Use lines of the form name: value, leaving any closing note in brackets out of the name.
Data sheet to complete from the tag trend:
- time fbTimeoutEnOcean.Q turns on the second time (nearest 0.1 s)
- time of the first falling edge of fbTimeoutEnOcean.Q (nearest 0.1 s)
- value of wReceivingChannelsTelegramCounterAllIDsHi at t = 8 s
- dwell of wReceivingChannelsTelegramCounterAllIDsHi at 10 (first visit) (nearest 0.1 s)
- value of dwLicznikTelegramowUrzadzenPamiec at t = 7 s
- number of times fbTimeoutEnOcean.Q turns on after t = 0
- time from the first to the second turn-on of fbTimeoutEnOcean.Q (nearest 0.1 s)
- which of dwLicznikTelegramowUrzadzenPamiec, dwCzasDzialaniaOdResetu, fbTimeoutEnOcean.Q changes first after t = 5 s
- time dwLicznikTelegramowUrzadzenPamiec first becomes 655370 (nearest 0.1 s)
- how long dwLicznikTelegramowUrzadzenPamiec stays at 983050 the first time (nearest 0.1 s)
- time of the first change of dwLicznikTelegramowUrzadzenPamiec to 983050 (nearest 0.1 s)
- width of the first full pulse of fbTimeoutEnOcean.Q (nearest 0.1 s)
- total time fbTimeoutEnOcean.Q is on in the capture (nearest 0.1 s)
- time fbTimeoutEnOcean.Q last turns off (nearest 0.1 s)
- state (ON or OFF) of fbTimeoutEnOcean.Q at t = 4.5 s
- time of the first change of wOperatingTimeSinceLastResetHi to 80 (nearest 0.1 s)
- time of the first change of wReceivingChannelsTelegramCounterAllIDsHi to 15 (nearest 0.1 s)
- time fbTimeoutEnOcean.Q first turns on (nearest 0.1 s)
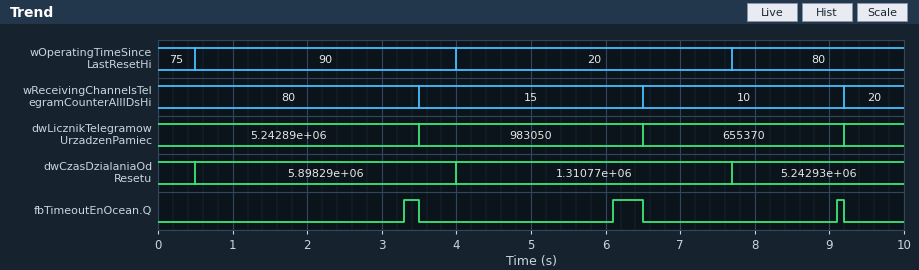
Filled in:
time fbTimeoutEnOcean.Q turns on the second time: 6.1 s
time of the first falling edge of fbTimeoutEnOcean.Q: 3.5 s
value of wReceivingChannelsTelegramCounterAllIDsHi at t = 8 s: 10
dwell of wReceivingChannelsTelegramCounterAllIDsHi at 10 (first visit): 2.7 s
value of dwLicznikTelegramowUrzadzenPamiec at t = 7 s: 655370
number of times fbTimeoutEnOcean.Q turns on after t = 0: 3
time from the first to the second turn-on of fbTimeoutEnOcean.Q: 2.8 s
which of dwLicznikTelegramowUrzadzenPamiec, dwCzasDzialaniaOdResetu, fbTimeoutEnOcean.Q changes first after t = 5 s: fbTimeoutEnOcean.Q
time dwLicznikTelegramowUrzadzenPamiec first becomes 655370: 6.5 s
how long dwLicznikTelegramowUrzadzenPamiec stays at 983050 the first time: 3.0 s
time of the first change of dwLicznikTelegramowUrzadzenPamiec to 983050: 3.5 s
width of the first full pulse of fbTimeoutEnOcean.Q: 0.2 s
total time fbTimeoutEnOcean.Q is on in the capture: 0.7 s
time fbTimeoutEnOcean.Q last turns off: 9.2 s
state (ON or OFF) of fbTimeoutEnOcean.Q at t = 4.5 s: OFF
time of the first change of wOperatingTimeSinceLastResetHi to 80: 7.7 s
time of the first change of wReceivingChannelsTelegramCounterAllIDsHi to 15: 3.5 s
time fbTimeoutEnOcean.Q first turns on: 3.3 s
